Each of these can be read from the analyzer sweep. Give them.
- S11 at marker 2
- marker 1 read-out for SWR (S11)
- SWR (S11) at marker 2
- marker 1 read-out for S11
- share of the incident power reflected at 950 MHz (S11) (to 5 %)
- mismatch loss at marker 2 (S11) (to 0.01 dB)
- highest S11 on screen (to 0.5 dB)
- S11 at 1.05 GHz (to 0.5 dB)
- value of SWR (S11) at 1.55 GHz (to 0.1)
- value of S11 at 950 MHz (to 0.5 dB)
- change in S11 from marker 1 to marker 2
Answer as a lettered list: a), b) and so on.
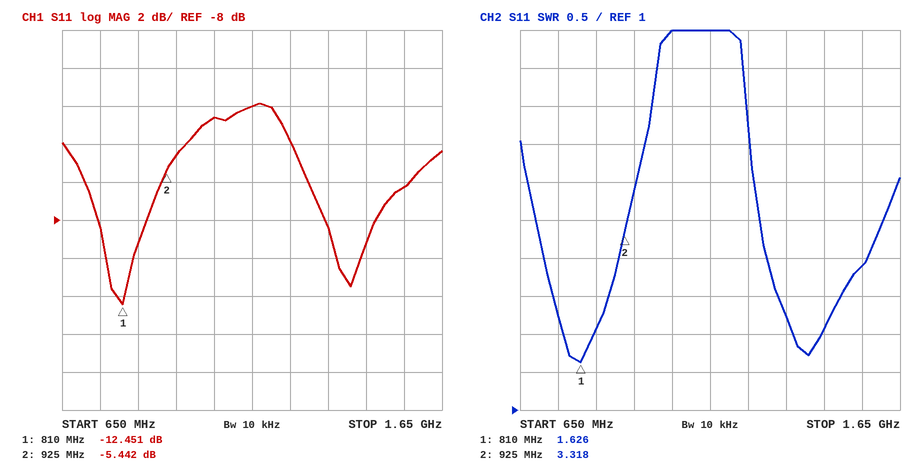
a) -5.442 dB
b) 1.626
c) 3.318
d) -12.451 dB
e) 35 %
f) 1.46 dB
g) -2.0 dB
h) -2.5 dB
i) 2.9
j) -4.5 dB
k) 7.009 dB
